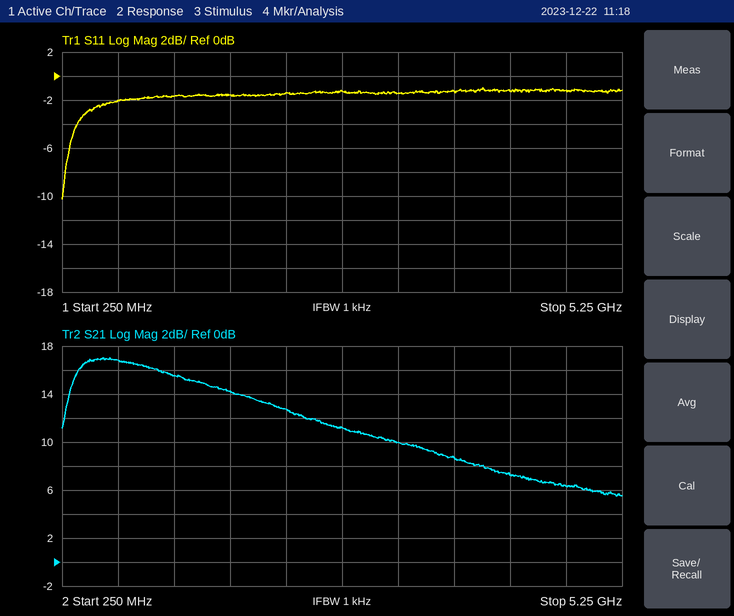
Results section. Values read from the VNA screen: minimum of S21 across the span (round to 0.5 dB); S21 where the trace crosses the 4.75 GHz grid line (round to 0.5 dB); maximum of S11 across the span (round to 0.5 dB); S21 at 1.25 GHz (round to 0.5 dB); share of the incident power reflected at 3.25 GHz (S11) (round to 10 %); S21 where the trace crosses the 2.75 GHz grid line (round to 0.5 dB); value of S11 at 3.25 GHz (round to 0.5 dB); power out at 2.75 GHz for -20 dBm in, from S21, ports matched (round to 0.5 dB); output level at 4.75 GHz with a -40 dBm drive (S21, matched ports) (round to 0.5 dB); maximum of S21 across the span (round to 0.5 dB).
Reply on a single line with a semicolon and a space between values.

5.5 dB; 6.5 dB; -1.0 dB; 15.5 dB; 70 %; 11.0 dB; -1.5 dB; -9.0 dBm; -33.5 dBm; 17.0 dB
